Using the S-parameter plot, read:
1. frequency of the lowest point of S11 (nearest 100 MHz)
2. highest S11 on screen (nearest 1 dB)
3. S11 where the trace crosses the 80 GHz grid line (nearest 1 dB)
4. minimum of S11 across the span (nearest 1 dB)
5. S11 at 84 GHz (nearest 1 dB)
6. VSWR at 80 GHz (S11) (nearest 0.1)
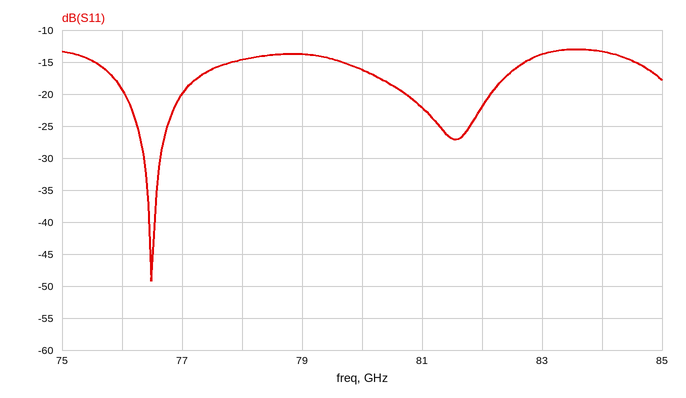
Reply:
76.5 GHz
-13 dB
-16 dB
-49 dB
-13 dB
1.4
